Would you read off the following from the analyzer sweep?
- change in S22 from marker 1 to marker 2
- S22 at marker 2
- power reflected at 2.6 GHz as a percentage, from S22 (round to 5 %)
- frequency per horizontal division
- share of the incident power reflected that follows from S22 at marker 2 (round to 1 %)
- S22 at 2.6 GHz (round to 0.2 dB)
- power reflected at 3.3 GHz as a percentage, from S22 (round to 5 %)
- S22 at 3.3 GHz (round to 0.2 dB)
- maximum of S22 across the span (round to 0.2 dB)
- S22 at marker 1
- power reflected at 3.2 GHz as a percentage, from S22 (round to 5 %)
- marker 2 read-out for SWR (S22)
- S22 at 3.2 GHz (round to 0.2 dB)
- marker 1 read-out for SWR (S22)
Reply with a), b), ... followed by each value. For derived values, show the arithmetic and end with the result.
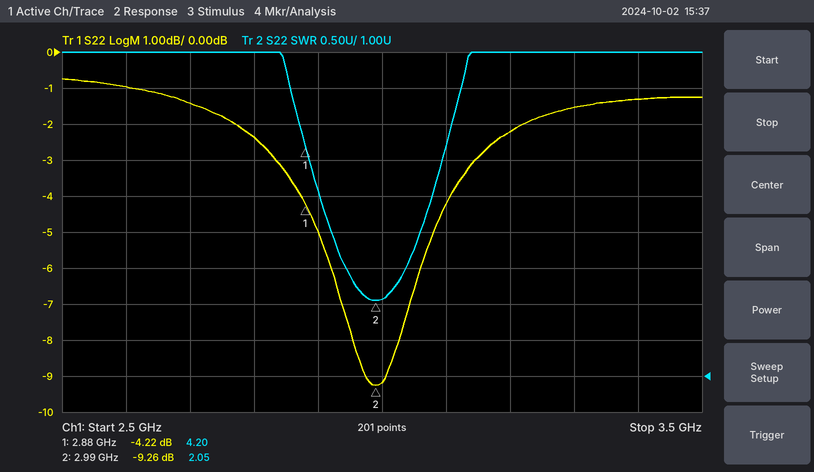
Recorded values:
a) -9.26 − (-4.22) = -5.04 dB
b) -9.26 dB
c) 10^(-1/10) ≈ 79.4 %, so 80 % to the nearest 5 %
d) 100 MHz
e) 10^(-9.26/10) ≈ 12 %
f) -1.0 dB
g) 10^(-1.6/10) ≈ 69.2 %, so 70 % to the nearest 5 %
h) -1.6 dB
i) -0.8 dB
j) -4.22 dB
k) 10^(-2.2/10) ≈ 60 %
l) 2.05
m) -2.2 dB
n) 4.20
